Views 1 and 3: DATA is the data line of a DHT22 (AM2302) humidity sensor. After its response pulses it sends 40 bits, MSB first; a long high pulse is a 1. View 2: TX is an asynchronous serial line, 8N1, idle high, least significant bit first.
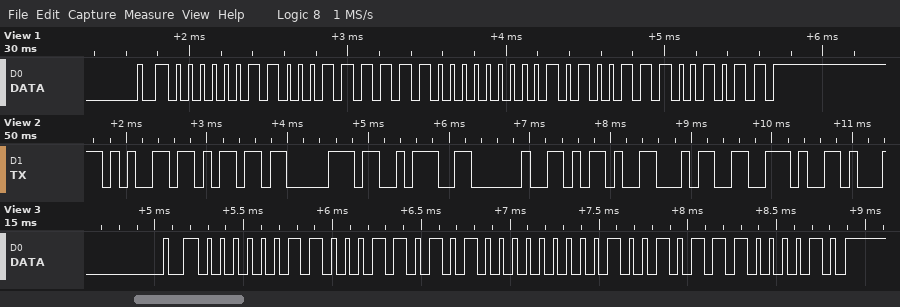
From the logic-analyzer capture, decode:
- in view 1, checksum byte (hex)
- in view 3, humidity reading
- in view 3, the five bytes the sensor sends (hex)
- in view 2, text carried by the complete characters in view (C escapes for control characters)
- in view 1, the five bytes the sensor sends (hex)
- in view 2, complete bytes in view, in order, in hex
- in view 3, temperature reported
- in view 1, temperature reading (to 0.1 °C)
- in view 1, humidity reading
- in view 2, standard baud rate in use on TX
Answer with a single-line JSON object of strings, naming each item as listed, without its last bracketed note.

{"in view 1, checksum byte": "0xCB", "in view 3, humidity reading": "79.4 %", "in view 3, the five bytes the sensor sends": "03 1A 80 25 C2", "in view 2, text carried by the complete characters in view": "\"emp: -4.\"", "in view 1, the five bytes the sensor sends": "03 1F 80 29 CB", "in view 2, complete bytes in view, in order, in hex": "0x65 0x6D 0x70 0x3A 0x20 0x2D 0x34 0x2E", "in view 3, temperature reported": "-3.7 °C", "in view 1, temperature reading": "-4.1 °C", "in view 1, humidity reading": "79.9 %", "in view 2, standard baud rate in use on TX": "9600 baud"}
